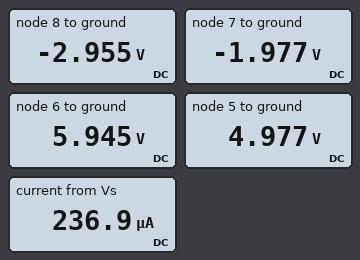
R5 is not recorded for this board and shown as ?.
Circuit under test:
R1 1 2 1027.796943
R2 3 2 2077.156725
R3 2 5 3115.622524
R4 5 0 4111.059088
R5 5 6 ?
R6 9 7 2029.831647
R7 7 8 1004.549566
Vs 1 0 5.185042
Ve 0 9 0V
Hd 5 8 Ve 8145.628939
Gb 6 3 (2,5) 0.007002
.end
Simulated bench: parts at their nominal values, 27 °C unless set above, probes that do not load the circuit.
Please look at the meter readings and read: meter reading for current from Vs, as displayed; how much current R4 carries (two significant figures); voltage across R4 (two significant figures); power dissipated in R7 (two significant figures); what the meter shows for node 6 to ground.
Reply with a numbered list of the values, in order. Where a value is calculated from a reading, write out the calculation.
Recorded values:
1. 236.9 µA
2. (4.977 V) / 4.111 kΩ = 1.2 mA
3. 4.977 V = 5.0 V
4. (-1.977 V - (-2.955 V))^2 / 1.005 kΩ = 950 µW
5. 5.945 V
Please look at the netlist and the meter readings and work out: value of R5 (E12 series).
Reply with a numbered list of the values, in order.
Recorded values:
1. 3.9 kΩ
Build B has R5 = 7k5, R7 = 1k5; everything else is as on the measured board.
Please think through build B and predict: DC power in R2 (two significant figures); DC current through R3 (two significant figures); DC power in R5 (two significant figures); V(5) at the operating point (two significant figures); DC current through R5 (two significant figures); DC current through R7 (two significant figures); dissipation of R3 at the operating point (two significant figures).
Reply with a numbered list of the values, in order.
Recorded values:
1. 41 µW
2. 6.5 µA
3. 150 µW
4. 5.1 V
5. 140 µA
6. 1.1 mA
7. 130 nW
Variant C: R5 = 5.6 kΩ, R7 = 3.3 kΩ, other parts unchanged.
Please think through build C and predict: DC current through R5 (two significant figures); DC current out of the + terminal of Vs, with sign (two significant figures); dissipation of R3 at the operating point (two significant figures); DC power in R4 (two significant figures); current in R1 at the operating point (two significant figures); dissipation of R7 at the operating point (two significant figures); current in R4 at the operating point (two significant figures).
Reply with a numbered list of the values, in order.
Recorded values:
1. 670 µA
2. -640 µA
3. 3.0 µW
4. 8.0 mW
5. 640 µA
6. 14 mW
7. 1.4 mA
